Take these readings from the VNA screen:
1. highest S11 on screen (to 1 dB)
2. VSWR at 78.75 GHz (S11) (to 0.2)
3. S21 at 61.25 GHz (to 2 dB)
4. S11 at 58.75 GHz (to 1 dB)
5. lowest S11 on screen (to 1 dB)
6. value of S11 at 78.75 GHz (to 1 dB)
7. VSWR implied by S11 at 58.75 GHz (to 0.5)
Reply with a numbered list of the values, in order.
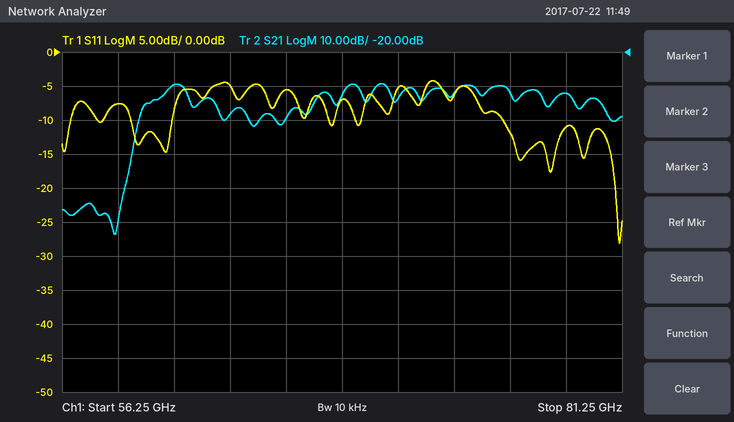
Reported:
1. -4 dB
2. 1.8
3. -30 dB
4. -8 dB
5. -28 dB
6. -11 dB
7. 2.5
